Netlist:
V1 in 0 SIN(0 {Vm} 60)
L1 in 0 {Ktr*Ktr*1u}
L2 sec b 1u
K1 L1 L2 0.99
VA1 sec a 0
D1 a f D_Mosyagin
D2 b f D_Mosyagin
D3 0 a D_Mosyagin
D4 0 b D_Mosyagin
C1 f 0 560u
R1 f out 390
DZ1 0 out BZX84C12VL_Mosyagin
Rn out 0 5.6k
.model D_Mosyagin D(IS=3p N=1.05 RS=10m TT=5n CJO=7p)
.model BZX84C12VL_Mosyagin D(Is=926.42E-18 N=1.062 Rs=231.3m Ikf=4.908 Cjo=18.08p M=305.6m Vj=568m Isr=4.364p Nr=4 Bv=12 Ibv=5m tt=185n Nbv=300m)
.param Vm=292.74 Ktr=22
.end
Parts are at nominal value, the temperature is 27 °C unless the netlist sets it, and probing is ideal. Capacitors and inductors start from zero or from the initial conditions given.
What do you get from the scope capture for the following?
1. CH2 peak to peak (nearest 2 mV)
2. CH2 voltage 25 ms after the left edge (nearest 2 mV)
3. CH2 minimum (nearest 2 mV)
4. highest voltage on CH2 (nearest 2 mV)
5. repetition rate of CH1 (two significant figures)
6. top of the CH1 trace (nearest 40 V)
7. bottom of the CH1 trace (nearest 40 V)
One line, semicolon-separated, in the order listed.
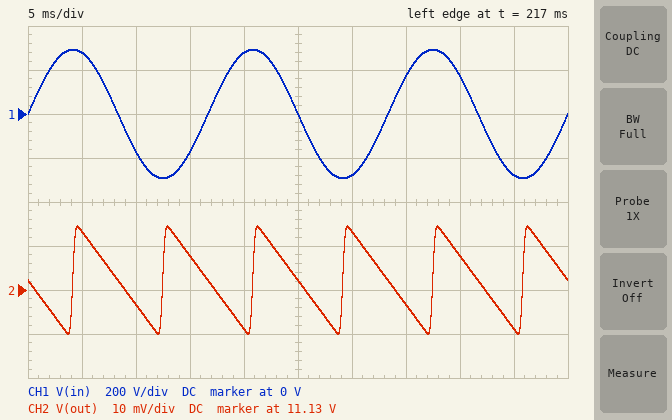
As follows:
24 mV; 11.132 V; 11.120 V; 11.144 V; 60 Hz; 280 V; -280 V
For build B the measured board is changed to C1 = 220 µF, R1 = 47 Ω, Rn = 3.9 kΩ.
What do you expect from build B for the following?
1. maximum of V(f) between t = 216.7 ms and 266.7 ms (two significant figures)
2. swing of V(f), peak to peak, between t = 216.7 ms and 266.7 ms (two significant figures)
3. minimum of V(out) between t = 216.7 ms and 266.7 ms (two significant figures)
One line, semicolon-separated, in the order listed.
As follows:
12 V; 100 mV; 12 V
